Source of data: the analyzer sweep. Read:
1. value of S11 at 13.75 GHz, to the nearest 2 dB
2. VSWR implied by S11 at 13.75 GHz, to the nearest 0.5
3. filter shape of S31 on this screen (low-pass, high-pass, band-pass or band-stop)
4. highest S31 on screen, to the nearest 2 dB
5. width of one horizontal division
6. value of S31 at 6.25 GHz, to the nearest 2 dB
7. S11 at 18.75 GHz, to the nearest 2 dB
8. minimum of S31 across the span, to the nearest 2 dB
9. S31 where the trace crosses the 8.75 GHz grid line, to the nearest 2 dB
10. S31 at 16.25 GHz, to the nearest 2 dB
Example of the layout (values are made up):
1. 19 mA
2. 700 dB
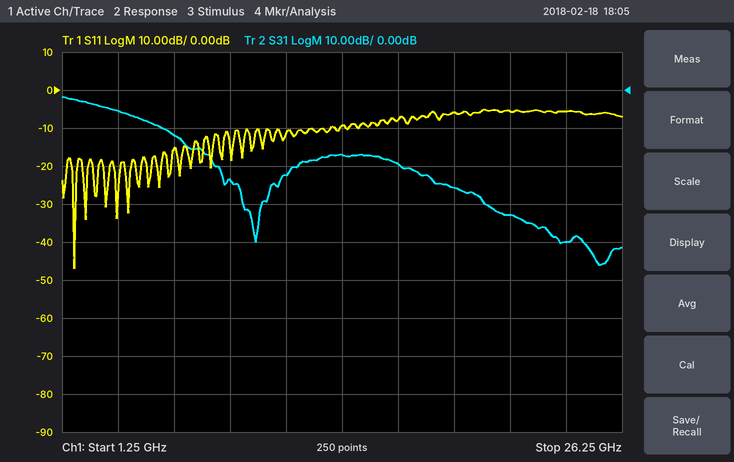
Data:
1. -10 dB
2. 2.0
3. low-pass
4. -2 dB
5. 2.5 GHz
6. -12 dB
7. -6 dB
8. -46 dB
9. -24 dB
10. -20 dB
